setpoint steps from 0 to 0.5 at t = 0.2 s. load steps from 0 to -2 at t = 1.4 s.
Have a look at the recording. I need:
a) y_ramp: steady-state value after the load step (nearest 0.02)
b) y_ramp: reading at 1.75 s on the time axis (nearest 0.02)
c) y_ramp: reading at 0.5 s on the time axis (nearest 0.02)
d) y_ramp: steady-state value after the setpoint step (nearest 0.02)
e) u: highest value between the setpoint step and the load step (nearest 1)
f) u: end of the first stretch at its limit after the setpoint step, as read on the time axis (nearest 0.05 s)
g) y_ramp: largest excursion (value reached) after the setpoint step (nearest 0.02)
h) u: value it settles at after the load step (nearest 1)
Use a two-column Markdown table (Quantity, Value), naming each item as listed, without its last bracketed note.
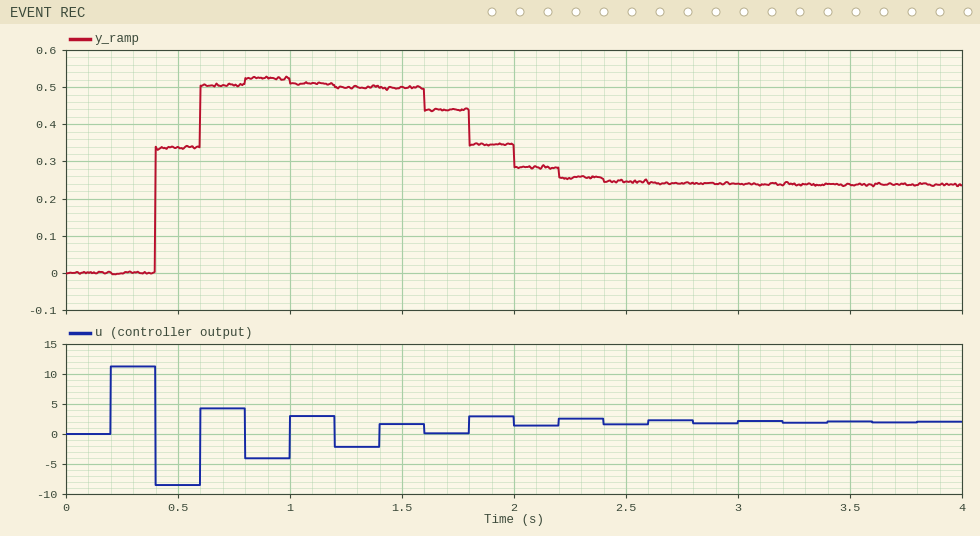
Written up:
| Quantity | Value |
|---|---|
| y_ramp: steady-state value after the load step | 0.24 |
| y_ramp: reading at 1.75 s on the time axis | 0.44 |
| y_ramp: reading at 0.5 s on the time axis | 0.34 |
| y_ramp: steady-state value after the setpoint step | 0.50 |
| u: highest value between the setpoint step and the load step | 11 |
| u: end of the first stretch at its limit after the setpoint step, as read on the time axis | 0.40 s |
| y_ramp: largest excursion (value reached) after the setpoint step | 0.52 |
| u: value it settles at after the load step | 2 |
